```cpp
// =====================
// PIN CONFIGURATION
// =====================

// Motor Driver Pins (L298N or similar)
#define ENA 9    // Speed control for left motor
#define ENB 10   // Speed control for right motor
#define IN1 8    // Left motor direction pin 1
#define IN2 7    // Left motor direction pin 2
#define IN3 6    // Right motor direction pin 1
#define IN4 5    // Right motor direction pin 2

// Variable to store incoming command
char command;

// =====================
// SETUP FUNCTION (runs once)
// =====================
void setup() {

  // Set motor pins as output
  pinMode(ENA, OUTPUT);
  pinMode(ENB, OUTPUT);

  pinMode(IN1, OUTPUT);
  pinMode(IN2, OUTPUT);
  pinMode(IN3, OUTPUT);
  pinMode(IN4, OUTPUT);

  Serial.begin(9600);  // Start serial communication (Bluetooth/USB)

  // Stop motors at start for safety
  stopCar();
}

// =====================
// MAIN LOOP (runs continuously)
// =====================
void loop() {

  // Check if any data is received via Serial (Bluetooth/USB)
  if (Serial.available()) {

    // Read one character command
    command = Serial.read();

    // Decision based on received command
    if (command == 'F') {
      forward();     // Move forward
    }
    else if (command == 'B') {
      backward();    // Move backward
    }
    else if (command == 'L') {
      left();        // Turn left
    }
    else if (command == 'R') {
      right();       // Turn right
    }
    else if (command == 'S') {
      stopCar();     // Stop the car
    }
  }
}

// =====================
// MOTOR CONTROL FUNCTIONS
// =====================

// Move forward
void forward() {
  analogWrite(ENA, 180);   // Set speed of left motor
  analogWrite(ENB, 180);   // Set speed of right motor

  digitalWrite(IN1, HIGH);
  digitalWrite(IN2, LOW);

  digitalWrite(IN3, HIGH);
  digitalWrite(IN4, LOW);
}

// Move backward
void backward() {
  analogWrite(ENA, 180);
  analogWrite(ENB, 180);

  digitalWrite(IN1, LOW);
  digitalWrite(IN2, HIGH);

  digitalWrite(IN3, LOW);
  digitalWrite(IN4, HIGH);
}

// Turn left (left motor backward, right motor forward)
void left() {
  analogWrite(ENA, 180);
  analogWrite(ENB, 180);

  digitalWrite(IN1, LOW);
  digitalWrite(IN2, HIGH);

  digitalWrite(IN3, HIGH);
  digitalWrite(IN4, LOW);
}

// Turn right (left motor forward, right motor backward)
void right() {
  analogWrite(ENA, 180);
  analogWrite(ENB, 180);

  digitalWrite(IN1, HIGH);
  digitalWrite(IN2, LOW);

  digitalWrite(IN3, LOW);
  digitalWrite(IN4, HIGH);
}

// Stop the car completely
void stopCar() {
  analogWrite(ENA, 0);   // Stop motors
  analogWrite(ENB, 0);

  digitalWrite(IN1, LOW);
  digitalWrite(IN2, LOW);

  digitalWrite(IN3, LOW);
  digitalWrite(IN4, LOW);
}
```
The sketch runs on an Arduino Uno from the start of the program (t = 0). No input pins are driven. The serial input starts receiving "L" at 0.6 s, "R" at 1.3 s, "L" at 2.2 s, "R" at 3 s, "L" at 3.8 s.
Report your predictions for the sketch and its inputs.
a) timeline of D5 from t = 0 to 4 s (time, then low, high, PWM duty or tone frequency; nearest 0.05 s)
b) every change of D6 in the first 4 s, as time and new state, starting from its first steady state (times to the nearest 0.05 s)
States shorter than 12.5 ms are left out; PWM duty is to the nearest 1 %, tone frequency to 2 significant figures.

0 s low; 1.3 s high; 2.2 s low; 3 s high; 3.8 s low
0 s low; 0.6 s high; 1.3 s low; 2.2 s high; 3 s low; 3.8 s high
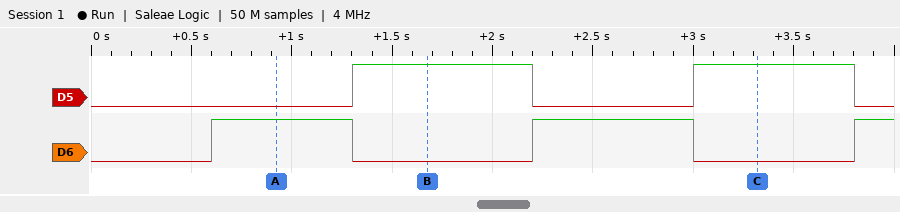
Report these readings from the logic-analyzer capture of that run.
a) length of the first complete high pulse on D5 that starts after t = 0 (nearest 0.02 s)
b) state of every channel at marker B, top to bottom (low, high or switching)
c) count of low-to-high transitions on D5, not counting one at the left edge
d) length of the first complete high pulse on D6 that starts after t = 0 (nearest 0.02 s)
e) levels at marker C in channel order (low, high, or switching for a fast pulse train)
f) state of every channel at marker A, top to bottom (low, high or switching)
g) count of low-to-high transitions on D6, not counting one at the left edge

0.90 s
D5 high, D6 low
2
0.70 s
D5 high, D6 low
D5 low, D6 high
3
